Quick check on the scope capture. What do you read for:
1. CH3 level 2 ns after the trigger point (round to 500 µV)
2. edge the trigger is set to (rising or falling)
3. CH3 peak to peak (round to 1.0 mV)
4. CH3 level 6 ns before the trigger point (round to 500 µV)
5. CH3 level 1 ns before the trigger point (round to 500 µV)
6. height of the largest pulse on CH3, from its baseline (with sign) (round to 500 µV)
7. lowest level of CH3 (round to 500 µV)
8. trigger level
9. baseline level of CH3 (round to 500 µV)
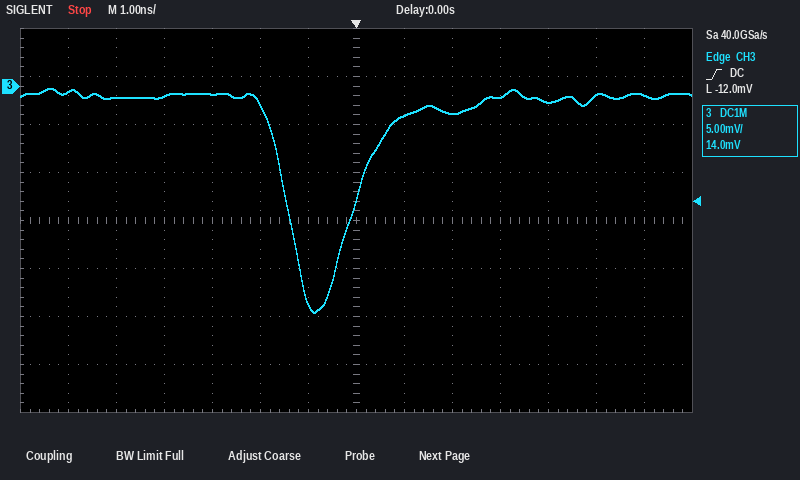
-3.0 mV
rising
23.0 mV
-500 µV
-22.5 mV
-22.5 mV
-23.5 mV
-12.0 mV
-1.0 mV
